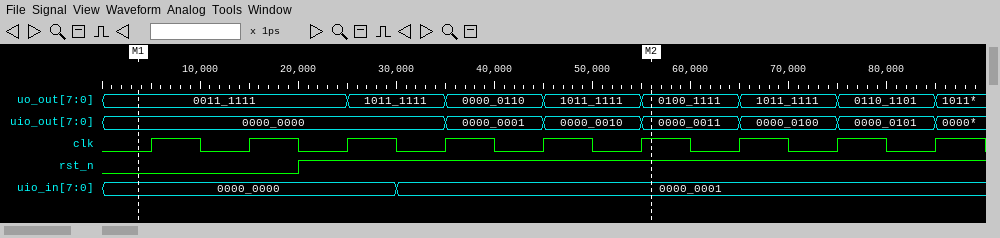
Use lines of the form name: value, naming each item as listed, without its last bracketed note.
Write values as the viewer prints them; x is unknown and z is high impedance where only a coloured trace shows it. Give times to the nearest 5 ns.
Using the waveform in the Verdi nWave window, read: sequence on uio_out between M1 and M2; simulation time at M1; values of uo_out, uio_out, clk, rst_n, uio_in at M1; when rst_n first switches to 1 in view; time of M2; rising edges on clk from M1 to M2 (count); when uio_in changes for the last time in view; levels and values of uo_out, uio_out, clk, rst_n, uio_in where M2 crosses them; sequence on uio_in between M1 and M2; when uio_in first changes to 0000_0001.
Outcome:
sequence on uio_out between M1 and M2: 0000_0000, 0000_0001, 0000_0010, 0000_0011
simulation time at M1: 5 ns
values of uo_out, uio_out, clk, rst_n, uio_in at M1: uo_out=0011_1111, uio_out=0000_0000, clk=0, rst_n=0, uio_in=0000_0000
when rst_n first switches to 1 in view: 20 ns
time of M2: 55 ns
rising edges on clk from M1 to M2: 6
when uio_in changes for the last time in view: 30 ns
levels and values of uo_out, uio_out, clk, rst_n, uio_in where M2 crosses them: uo_out=0100_1111, uio_out=0000_0011, clk=1, rst_n=1, uio_in=0000_0001
sequence on uio_in between M1 and M2: 0000_0000, 0000_0001
when uio_in first changes to 0000_0001: 30 ns
